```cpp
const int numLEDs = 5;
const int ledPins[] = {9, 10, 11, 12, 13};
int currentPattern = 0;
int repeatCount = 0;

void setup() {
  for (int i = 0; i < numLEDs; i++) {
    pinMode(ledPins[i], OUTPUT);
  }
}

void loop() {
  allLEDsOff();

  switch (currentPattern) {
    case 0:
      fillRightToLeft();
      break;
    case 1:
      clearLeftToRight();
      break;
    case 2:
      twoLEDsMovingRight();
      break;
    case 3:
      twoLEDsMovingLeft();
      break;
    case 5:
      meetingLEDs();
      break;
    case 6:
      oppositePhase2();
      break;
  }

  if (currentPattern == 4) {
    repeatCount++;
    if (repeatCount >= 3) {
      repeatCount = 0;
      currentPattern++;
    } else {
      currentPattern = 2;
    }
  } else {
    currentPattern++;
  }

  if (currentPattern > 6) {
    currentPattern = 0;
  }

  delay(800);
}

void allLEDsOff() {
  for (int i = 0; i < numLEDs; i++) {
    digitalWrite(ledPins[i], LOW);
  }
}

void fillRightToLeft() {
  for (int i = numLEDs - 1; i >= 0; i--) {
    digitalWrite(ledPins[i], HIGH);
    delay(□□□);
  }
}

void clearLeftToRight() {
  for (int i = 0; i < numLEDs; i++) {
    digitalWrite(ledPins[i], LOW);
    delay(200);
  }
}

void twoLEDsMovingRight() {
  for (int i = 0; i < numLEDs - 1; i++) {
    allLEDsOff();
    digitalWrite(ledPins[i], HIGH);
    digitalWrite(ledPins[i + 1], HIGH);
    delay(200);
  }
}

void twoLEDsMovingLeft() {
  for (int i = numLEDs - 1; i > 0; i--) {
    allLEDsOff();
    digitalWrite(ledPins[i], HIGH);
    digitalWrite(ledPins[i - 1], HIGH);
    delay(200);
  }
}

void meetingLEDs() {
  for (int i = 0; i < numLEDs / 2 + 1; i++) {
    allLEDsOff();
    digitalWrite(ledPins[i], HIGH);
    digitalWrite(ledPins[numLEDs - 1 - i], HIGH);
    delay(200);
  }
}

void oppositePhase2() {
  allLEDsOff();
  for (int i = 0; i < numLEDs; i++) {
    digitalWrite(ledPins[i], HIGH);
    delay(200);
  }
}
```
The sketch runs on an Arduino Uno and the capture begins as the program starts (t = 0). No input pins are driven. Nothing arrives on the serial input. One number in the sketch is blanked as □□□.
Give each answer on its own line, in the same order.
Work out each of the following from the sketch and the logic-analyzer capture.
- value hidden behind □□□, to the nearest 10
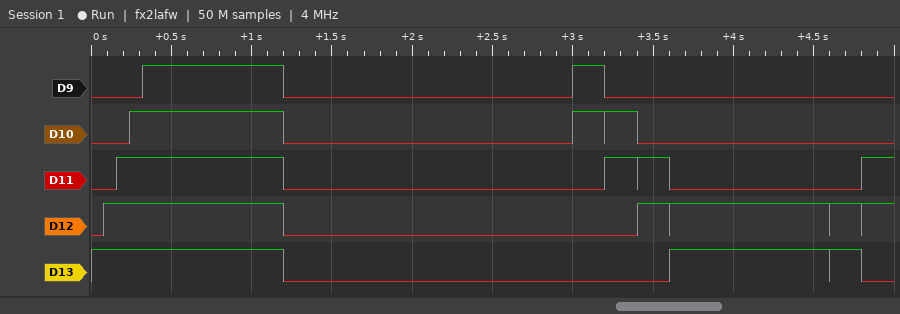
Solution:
80
